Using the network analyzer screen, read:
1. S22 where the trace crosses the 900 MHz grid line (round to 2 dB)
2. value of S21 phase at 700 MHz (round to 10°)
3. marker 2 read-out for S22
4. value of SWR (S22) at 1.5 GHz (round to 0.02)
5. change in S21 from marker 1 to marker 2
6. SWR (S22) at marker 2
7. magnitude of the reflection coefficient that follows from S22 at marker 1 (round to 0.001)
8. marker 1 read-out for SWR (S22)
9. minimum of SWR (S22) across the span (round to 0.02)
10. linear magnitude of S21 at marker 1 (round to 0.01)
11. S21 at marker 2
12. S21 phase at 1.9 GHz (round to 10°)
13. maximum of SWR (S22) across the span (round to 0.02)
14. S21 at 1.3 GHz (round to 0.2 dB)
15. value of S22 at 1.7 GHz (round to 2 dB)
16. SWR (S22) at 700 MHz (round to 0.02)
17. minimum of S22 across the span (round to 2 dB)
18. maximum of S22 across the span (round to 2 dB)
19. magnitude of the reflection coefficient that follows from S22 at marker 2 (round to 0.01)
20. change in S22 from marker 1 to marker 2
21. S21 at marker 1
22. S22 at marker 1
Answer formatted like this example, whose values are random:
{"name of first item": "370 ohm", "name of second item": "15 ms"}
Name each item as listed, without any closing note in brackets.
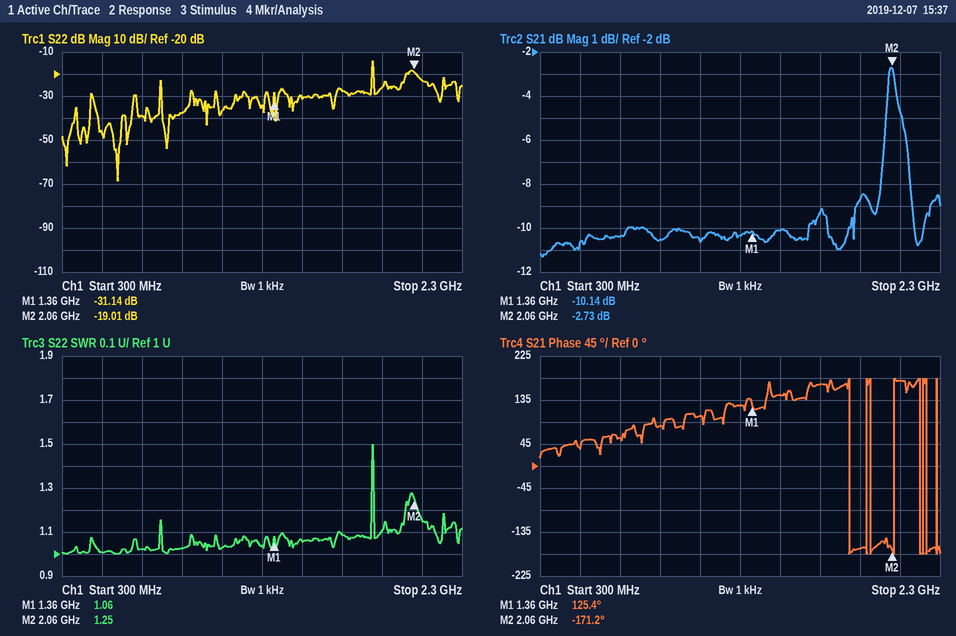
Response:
{"S22 where the trace crosses the 900 MHz grid line": "-38 dB", "value of S21 phase at 700 MHz": "60°", "marker 2 read-out for S22": "-19.01 dB", "value of SWR (S22) at 1.5 GHz": "1.06", "change in S21 from marker 1 to marker 2": "7.41 dB", "SWR (S22) at marker 2": "1.25", "magnitude of the reflection coefficient that follows from S22 at marker 1": "0.028", "marker 1 read-out for SWR": "1.06", "minimum of SWR (S22) across the span": "1.00", "linear magnitude of S21 at marker 1": "0.31", "S21 at marker 2": "-2.73 dB", "S21 phase at 1.9 GHz": "-170°", "maximum of SWR (S22) across the span": "1.50", "S21 at 1.3 GHz": "-10.4 dB", "value of S22 at 1.7 GHz": "-28 dB", "SWR (S22) at 700 MHz": "1.02", "minimum of S22 across the span": "-68 dB", "maximum of S22 across the span": "-14 dB", "magnitude of the reflection coefficient that follows from S22 at marker 2": "0.11", "change in S22 from marker 1 to marker 2": "12.13 dB", "S21 at marker 1": "-10.14 dB", "S22 at marker 1": "-31.14 dB"}
